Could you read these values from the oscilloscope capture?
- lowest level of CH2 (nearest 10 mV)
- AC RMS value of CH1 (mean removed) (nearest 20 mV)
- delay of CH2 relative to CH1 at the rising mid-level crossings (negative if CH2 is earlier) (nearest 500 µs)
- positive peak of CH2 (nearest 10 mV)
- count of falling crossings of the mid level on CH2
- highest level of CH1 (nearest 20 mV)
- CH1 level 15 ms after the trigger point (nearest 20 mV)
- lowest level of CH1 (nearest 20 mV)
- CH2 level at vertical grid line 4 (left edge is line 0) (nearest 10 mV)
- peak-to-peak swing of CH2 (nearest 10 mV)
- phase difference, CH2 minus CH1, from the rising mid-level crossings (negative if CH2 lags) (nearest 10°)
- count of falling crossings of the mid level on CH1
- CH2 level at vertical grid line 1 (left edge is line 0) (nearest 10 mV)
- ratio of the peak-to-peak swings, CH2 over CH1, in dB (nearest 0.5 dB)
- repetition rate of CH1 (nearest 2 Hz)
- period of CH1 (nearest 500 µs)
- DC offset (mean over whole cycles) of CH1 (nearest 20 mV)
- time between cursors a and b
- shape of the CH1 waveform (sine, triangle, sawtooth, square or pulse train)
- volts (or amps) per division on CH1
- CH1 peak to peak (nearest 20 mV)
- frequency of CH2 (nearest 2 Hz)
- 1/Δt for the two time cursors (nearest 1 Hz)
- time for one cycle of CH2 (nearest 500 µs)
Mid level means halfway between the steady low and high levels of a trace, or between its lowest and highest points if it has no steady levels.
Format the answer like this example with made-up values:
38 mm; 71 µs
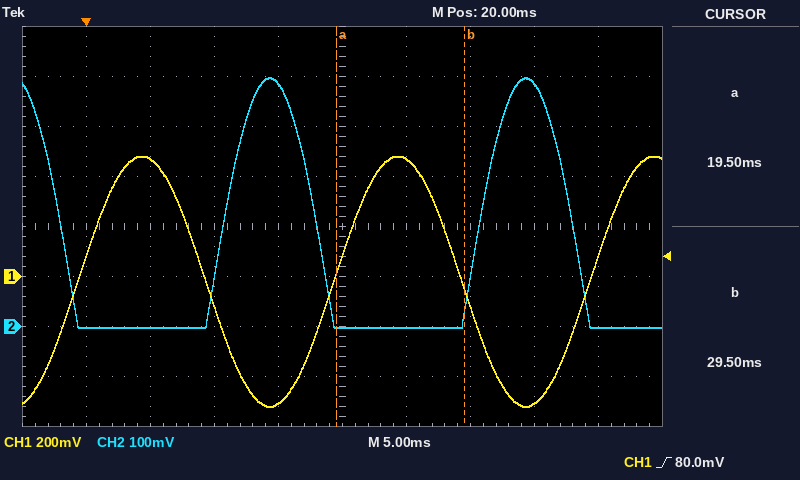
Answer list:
0 mV; 360 mV; -8.5 ms; 500 mV; 3; 480 mV; -500 mV; -520 mV; 490 mV; 500 mV; +150°; 2; 0 mV; -6.0 dB; 50 Hz; 20.0 ms; -20 mV; 10.0 ms; sine; 200 mV; 1.00 V; 50 Hz; 100 Hz; 20.0 ms
